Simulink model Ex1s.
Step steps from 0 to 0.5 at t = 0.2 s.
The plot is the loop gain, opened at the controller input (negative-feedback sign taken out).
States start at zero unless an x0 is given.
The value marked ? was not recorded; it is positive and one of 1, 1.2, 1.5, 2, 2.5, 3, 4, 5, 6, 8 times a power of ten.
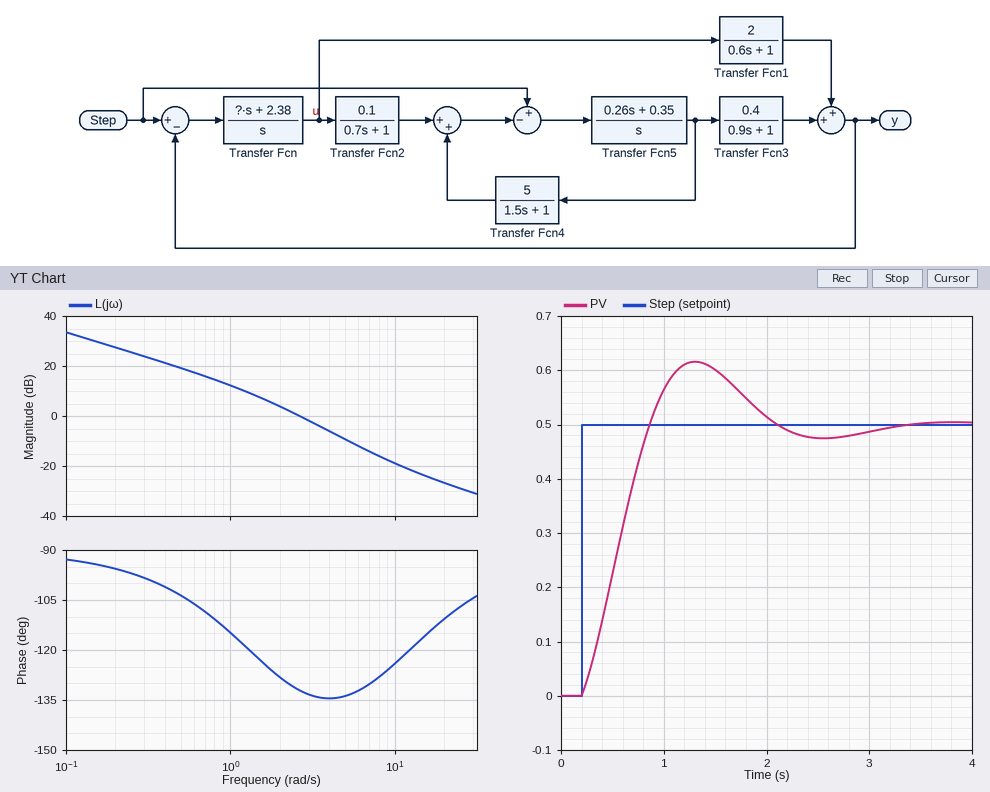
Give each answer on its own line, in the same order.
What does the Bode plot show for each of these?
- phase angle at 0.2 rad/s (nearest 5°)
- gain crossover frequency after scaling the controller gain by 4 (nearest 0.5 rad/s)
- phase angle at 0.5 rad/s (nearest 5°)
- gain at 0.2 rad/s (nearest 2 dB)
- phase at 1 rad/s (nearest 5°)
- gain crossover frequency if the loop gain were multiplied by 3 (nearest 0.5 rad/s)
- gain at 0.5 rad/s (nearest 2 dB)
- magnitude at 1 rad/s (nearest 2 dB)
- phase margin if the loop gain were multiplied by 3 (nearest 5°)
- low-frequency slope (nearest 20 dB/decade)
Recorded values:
-95°
6.0 rad/s
-105°
28 dB
-115°
5.0 rad/s
20 dB
12 dB
45°
-20 dB/decade
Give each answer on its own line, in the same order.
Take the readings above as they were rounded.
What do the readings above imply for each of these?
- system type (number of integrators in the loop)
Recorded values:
1
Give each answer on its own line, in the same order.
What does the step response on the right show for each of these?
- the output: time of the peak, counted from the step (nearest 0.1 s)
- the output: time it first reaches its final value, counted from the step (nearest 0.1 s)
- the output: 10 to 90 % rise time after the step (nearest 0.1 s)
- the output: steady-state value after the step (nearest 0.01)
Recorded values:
1.1 s
0.7 s
0.5 s
0.50
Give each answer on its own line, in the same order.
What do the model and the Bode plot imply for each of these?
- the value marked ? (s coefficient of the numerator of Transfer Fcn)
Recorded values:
0.25
